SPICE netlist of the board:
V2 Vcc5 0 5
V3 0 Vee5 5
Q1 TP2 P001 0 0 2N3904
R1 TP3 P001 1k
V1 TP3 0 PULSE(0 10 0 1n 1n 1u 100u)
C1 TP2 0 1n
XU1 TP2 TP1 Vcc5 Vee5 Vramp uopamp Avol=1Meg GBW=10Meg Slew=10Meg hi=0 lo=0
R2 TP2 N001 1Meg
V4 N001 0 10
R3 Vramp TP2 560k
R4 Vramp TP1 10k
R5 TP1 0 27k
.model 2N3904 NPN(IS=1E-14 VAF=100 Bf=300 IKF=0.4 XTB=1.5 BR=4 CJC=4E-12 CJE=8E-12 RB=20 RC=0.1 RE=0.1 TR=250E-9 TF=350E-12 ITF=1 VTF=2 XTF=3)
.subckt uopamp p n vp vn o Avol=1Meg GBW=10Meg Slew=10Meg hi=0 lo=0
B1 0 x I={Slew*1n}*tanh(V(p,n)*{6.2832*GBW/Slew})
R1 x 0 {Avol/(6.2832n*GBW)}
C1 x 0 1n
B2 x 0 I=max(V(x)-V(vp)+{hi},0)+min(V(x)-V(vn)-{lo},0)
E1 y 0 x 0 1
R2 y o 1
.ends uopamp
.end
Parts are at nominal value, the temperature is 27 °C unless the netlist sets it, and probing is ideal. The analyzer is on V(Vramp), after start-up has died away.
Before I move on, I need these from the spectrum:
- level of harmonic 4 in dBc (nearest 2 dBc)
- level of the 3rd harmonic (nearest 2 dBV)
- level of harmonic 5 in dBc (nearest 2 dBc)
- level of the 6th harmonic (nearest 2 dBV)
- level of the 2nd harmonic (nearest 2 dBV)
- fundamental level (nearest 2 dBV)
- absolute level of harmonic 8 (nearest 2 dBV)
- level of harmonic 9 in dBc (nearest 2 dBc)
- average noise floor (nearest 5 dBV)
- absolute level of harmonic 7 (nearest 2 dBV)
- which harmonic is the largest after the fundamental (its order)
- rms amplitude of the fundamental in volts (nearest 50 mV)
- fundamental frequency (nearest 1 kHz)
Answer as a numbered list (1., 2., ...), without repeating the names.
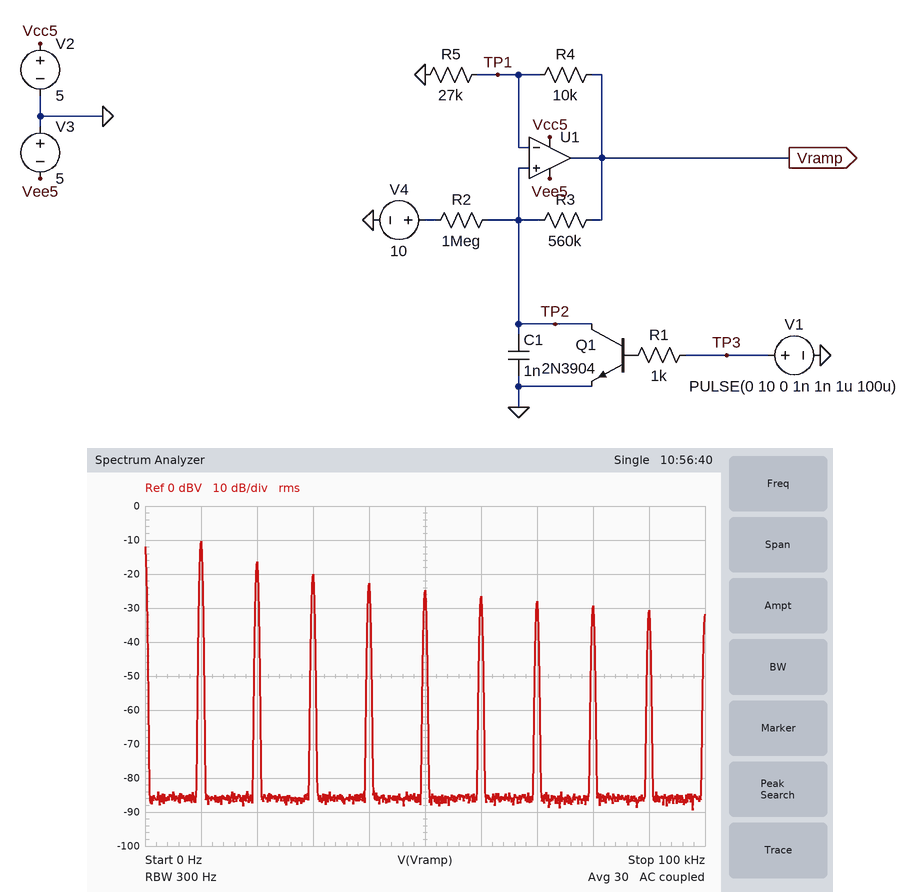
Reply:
1. -12 dBc
2. -20 dBV
3. -14 dBc
4. -26 dBV
5. -16 dBV
6. -10 dBV
7. -30 dBV
8. -20 dBc
9. -85 dBV
10. -28 dBV
11. 2
12. 300 mV
13. 10 kHz
